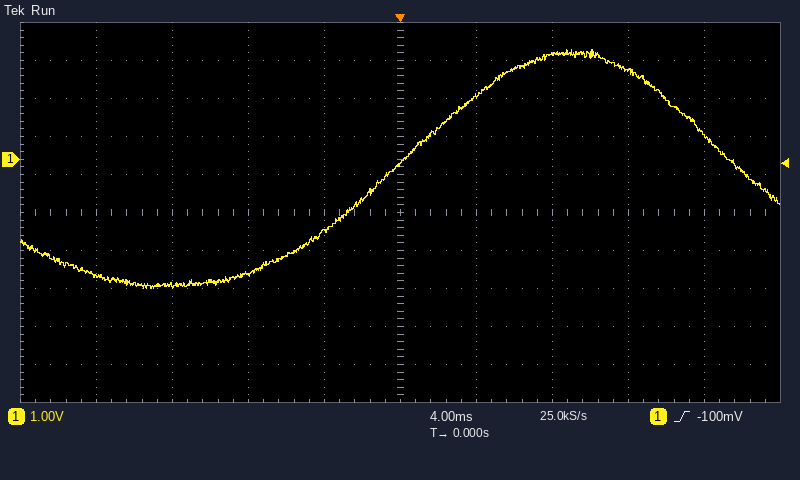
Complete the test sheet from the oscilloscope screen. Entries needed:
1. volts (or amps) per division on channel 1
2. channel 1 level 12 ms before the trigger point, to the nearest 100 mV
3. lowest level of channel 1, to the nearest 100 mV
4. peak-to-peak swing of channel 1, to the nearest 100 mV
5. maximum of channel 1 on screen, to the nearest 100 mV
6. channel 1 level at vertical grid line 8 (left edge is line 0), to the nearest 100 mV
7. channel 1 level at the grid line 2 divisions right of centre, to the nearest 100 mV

1 V
-3.3 V
-3.4 V
6.3 V
2.9 V
2.3 V
2.8 V
